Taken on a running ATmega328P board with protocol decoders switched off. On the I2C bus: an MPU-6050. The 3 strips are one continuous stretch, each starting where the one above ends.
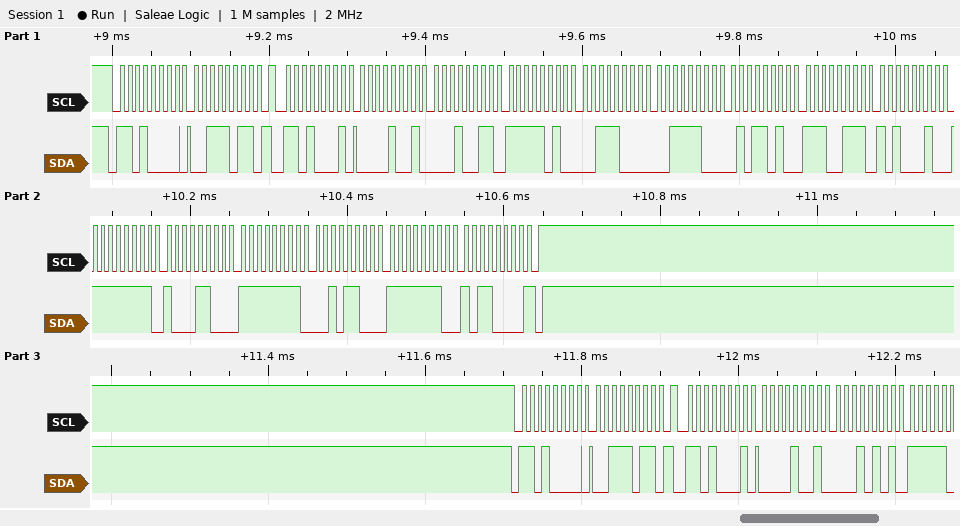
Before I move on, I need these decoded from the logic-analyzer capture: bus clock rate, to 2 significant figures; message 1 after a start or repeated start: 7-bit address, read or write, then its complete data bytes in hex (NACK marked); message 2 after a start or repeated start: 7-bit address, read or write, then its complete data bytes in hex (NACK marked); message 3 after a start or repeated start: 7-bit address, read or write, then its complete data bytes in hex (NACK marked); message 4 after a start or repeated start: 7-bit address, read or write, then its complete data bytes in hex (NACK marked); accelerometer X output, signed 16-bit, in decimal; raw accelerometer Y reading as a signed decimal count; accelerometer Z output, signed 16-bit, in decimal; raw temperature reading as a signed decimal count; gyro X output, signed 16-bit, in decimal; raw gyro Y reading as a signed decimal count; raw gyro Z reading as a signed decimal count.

100 kHz
0x68 write: 3B
0x68 read: 09 13 FA 38 3C 5A E7 A2 FF 8C FF 2C FE B0 NACK
0x68 write: 3B
0x68 read: 09 15
2323
-1480
15450
-6238
-116
-212
-336
